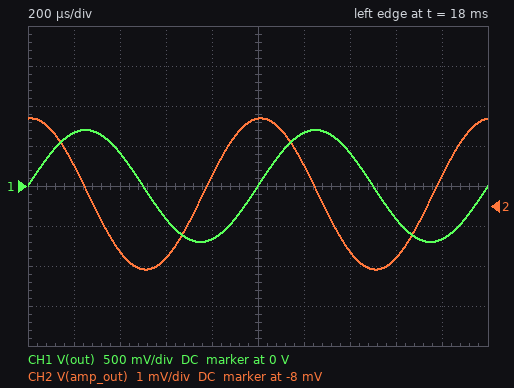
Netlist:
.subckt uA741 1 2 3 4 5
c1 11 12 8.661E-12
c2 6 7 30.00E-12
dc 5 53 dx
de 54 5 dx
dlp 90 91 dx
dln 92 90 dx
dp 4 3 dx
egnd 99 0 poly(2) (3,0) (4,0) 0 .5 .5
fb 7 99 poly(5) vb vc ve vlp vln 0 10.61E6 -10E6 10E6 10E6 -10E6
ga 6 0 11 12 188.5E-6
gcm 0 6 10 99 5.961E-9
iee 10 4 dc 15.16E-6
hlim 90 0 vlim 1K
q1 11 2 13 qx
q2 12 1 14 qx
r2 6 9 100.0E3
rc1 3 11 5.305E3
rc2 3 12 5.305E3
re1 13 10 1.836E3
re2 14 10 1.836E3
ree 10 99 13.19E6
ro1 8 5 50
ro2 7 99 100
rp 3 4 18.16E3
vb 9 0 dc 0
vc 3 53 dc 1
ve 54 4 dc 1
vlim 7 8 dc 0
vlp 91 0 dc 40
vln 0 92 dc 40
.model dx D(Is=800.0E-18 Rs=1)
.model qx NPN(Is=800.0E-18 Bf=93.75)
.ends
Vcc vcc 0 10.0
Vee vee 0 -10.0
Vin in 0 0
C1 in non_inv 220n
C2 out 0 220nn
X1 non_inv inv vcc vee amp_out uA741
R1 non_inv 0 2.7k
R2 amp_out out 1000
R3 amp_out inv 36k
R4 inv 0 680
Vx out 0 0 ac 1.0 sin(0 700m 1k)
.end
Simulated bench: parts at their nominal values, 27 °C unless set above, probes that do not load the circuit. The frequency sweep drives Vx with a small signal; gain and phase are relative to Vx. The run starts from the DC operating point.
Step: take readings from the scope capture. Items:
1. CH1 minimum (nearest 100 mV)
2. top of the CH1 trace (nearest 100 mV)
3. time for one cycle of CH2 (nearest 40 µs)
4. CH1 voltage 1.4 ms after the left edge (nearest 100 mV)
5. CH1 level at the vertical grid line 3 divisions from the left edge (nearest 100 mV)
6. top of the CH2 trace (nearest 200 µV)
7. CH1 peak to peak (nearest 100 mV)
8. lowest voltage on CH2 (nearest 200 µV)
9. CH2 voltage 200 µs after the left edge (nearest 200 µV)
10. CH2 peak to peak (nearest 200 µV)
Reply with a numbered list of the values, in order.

1. -700 mV
2. 700 mV
3. 1.00 ms
4. 400 mV
5. -400 mV
6. -5.8 mV
7. 1.4 V
8. -9.6 mV
9. -7.0 mV
10. 3.8 mV
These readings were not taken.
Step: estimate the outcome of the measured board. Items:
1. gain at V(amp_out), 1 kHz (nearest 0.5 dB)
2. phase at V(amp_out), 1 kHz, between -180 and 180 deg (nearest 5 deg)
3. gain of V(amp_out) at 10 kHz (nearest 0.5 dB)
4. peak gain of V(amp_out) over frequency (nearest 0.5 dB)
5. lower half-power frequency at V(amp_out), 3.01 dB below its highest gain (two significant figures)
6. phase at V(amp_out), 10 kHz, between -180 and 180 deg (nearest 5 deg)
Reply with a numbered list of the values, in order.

1. -51.5 dB
2. 85 deg
3. -32.5 dB
4. -26.5 dB
5. 18 kHz
6. 60 deg
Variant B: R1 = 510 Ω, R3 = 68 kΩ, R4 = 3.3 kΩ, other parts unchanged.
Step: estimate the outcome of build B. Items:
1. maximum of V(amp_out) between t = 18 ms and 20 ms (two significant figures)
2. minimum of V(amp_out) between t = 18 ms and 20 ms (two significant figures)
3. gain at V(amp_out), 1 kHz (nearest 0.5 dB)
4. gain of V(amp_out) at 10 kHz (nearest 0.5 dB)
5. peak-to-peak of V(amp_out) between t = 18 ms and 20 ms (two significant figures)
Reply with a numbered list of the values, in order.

1. 5.7 mV
2. 4.2 mV
3. -59.5 dB
4. -39.5 dB
5. 1.5 mV
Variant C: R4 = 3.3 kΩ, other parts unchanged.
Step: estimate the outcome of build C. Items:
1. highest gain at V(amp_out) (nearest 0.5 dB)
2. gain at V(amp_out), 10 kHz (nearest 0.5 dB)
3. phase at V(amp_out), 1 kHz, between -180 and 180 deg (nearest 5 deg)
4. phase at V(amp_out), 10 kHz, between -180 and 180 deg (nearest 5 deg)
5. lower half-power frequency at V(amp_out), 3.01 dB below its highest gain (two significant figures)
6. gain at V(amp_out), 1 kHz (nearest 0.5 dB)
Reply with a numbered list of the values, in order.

1. -26.0 dB
2. -44.5 dB
3. 90 deg
4. 85 deg
5. 81 kHz
6. -64.5 dB
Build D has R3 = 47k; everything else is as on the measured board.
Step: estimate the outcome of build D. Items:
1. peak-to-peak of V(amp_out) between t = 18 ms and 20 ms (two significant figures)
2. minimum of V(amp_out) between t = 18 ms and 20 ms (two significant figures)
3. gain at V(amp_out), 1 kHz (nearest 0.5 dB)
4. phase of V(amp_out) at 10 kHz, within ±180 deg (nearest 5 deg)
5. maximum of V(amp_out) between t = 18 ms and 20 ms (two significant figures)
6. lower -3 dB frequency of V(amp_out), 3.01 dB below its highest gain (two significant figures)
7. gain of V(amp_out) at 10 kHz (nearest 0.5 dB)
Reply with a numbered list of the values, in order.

1. 4.9 mV
2. -12 mV
3. -49.0 dB
4. 55 deg
5. -7.5 mV
6. 14 kHz
7. -31.0 dB
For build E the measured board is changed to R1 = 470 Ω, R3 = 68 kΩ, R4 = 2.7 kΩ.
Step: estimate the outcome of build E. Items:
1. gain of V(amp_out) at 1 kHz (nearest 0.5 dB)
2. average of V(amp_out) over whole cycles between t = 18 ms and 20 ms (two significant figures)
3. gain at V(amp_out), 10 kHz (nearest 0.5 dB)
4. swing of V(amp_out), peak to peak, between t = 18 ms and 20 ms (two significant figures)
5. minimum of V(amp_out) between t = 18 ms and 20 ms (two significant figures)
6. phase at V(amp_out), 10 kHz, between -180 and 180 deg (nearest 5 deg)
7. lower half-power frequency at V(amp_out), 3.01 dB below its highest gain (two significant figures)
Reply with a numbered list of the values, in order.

1. -57.5 dB
2. 4.9 mV
3. -38.0 dB
4. 1.8 mV
5. 4.0 mV
6. 75 deg
7. 37 kHz
